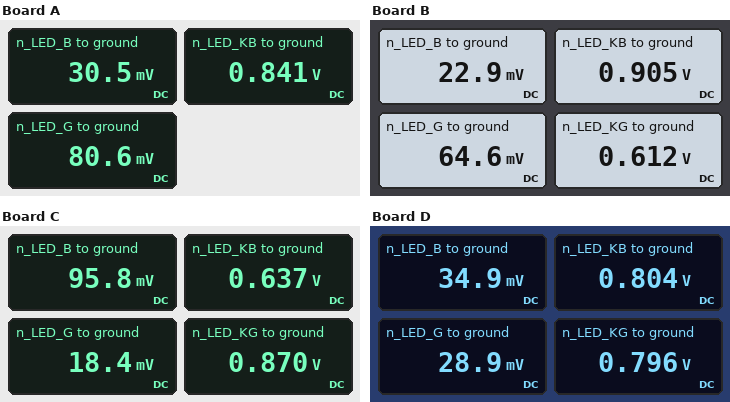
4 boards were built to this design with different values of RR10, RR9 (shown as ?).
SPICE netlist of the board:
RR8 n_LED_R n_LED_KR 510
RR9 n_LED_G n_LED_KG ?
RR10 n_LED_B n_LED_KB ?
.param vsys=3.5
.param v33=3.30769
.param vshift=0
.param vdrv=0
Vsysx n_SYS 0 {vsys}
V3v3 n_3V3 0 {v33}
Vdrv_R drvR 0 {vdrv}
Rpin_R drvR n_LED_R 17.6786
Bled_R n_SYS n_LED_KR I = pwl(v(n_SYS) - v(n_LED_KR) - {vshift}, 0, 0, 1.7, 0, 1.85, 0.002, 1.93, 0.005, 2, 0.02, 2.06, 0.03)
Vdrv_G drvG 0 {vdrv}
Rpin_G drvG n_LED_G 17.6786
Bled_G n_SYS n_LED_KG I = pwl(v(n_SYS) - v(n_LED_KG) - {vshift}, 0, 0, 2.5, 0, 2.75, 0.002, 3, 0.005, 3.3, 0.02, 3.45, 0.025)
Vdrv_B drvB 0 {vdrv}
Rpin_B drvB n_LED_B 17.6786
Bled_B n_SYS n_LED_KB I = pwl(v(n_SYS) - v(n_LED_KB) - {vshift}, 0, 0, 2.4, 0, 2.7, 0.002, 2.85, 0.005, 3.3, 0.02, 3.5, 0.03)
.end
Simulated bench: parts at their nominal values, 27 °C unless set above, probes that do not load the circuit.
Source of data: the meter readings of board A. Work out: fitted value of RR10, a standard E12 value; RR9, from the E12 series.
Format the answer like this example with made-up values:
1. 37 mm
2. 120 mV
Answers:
1. 470 Ω
2. 100 Ω
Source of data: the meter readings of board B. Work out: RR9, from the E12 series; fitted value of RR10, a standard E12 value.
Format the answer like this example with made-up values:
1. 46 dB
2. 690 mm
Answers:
1. 150 Ω
2. 680 Ω
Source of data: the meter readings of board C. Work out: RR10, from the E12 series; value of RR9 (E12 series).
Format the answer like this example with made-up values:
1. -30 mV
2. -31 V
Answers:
1. 100 Ω
2. 820 Ω
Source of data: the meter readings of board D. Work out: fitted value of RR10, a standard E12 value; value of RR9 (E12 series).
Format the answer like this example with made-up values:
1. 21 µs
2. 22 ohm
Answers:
1. 390 Ω
2. 470 Ω
